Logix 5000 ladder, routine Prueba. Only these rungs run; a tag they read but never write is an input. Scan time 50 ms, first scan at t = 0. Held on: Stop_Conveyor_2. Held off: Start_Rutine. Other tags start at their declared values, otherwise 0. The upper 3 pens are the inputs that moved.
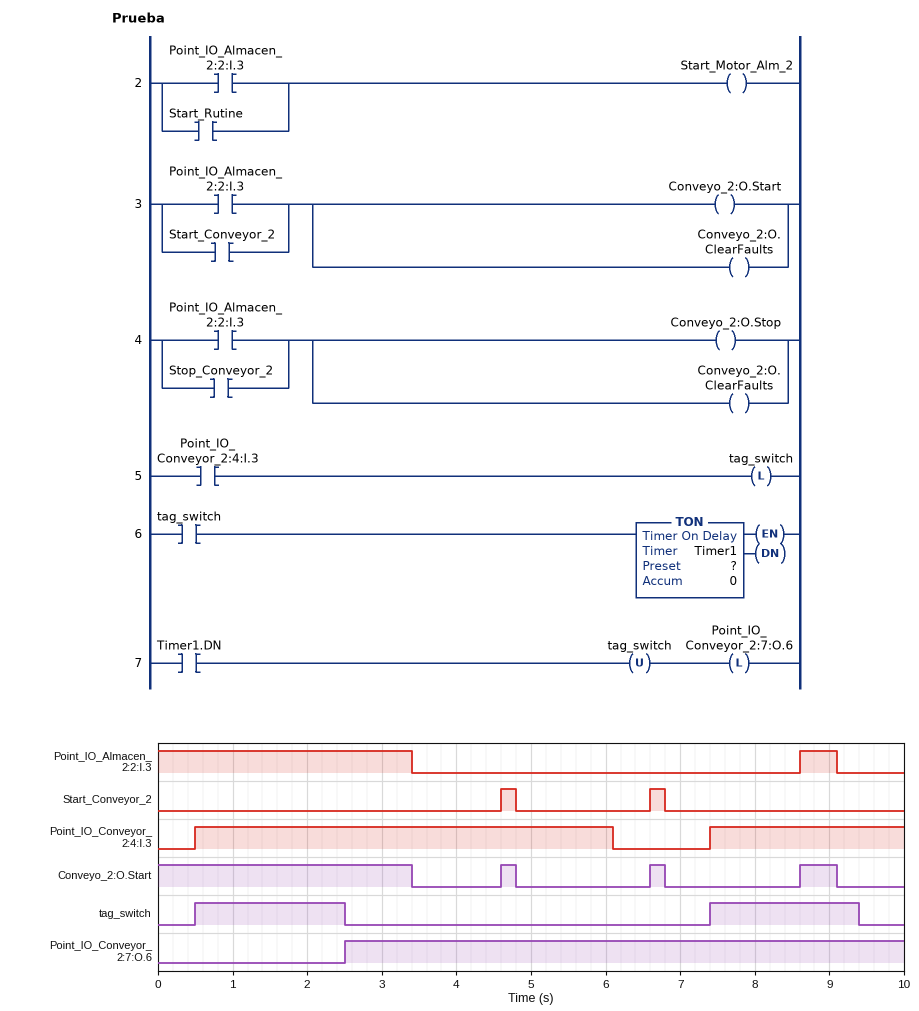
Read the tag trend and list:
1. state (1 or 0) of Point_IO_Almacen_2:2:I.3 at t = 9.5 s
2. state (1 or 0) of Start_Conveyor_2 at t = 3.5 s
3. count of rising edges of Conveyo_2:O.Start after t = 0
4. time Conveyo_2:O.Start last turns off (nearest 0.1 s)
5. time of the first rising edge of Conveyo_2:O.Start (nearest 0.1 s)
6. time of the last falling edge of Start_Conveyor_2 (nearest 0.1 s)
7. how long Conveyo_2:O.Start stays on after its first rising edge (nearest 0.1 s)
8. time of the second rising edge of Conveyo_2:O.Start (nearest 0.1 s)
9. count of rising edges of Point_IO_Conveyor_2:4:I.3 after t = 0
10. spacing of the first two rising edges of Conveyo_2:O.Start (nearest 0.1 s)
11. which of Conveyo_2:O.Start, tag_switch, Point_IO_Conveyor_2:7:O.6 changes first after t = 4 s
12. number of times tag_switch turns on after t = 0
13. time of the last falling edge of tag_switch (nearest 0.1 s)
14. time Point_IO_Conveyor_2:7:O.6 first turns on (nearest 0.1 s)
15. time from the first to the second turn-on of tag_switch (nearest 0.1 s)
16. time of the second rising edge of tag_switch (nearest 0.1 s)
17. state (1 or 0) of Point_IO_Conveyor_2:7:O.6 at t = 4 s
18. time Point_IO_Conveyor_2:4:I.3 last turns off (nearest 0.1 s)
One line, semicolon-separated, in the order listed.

0; 0; 3; 9.1 s; 4.6 s; 6.8 s; 0.2 s; 6.6 s; 2; 2.0 s; Conveyo_2:O.Start; 2; 9.4 s; 2.5 s; 6.9 s; 7.4 s; 1; 6.1 s
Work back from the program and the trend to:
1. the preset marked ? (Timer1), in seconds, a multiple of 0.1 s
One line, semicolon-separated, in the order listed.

2.0 s
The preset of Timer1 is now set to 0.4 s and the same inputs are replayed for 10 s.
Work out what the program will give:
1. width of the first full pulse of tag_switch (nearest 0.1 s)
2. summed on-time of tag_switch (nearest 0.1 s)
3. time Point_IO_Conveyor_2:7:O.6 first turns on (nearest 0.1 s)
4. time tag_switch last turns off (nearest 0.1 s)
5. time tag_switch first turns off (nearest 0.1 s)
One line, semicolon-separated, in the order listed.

0.4 s; 0.8 s; 0.9 s; 7.8 s; 0.9 s
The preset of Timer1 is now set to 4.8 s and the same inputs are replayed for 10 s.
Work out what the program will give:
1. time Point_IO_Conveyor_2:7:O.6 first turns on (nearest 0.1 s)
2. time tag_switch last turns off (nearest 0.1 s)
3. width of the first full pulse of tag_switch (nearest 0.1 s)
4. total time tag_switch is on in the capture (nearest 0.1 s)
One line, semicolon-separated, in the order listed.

5.3 s; 5.3 s; 4.8 s; 7.4 s
